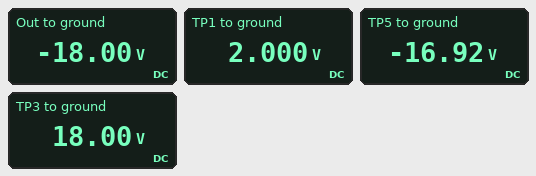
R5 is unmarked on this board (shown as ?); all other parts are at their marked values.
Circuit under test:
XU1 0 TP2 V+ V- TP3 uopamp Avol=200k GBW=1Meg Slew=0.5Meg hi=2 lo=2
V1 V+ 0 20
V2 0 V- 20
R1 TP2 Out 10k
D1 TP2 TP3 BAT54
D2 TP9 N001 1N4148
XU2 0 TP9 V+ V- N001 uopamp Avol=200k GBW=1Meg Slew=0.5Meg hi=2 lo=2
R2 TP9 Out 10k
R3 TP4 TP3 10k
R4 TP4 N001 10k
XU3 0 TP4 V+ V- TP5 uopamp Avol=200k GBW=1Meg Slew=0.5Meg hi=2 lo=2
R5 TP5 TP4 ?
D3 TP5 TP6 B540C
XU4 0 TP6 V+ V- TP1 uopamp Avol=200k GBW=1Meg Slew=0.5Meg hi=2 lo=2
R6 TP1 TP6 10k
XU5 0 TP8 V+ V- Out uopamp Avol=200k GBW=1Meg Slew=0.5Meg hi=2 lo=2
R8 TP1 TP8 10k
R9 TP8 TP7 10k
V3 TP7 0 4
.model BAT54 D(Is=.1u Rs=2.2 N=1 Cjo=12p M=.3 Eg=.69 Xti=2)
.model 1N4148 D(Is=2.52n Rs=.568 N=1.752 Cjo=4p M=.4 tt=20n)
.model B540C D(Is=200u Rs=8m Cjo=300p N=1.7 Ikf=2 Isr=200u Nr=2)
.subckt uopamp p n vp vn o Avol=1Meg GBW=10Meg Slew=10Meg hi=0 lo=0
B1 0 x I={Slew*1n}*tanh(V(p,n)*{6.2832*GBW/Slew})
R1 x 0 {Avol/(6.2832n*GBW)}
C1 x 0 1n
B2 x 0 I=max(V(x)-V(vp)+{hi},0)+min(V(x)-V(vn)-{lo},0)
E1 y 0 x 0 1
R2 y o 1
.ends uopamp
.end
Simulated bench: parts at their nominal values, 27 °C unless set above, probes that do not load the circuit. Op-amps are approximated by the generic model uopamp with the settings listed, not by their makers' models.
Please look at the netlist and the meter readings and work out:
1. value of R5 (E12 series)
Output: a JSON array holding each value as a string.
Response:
["4.7 kΩ"]
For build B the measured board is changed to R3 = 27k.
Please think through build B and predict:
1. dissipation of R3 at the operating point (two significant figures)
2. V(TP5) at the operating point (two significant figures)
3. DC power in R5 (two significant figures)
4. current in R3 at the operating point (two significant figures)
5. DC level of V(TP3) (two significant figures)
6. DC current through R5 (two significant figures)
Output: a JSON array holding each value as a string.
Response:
["12 mW", "-12 V", "29 mW", "670 µA", "18 V", "2.5 mA"]
